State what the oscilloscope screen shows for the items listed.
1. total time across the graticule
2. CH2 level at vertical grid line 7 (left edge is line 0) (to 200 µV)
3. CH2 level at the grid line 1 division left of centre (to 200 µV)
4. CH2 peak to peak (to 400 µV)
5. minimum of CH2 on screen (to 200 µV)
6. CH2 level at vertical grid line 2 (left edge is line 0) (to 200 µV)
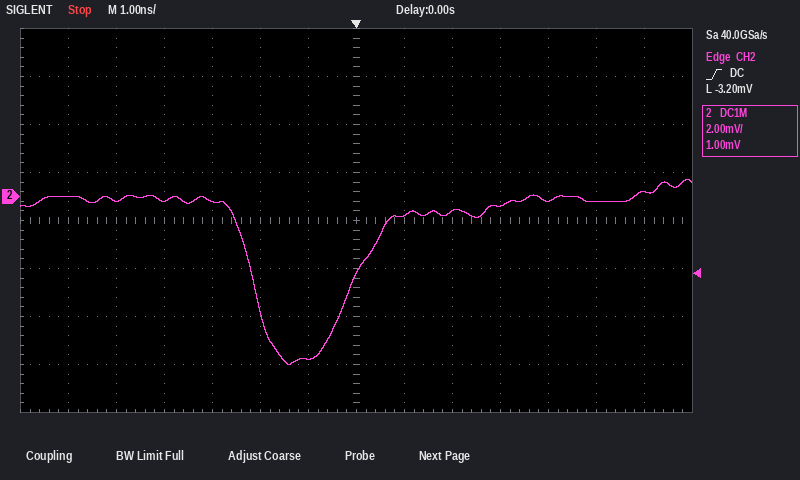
14 ns
-3.2 mV
-6.8 mV
7.6 mV
-7.0 mV
-200 µV
